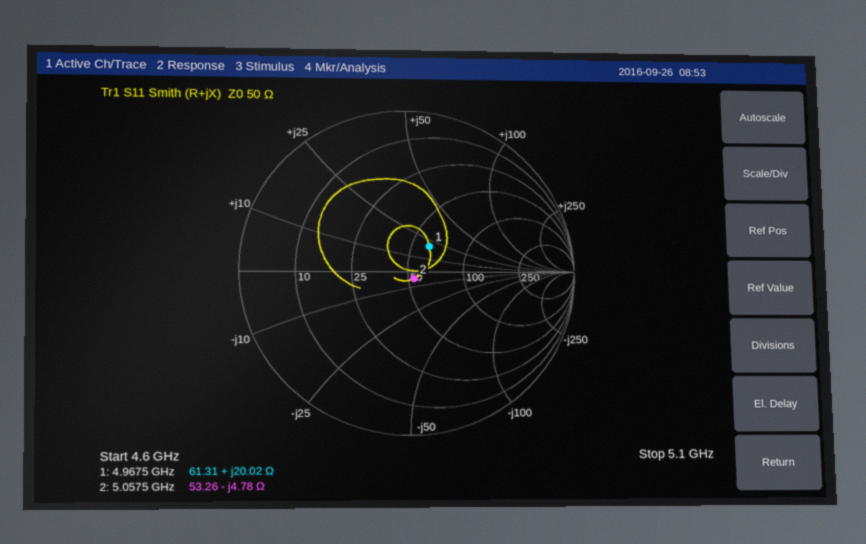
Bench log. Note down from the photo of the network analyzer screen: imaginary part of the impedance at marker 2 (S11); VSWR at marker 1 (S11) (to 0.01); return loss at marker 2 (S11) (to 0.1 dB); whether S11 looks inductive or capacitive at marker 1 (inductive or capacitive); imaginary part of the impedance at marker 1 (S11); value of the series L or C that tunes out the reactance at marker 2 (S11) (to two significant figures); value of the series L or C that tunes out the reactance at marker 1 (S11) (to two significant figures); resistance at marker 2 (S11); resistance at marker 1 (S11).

-4.78 Ω
1.51
25.0 dB
inductive
+20.02 Ω
150 pH
1.6 pF
53.26 Ω
61.31 Ω
